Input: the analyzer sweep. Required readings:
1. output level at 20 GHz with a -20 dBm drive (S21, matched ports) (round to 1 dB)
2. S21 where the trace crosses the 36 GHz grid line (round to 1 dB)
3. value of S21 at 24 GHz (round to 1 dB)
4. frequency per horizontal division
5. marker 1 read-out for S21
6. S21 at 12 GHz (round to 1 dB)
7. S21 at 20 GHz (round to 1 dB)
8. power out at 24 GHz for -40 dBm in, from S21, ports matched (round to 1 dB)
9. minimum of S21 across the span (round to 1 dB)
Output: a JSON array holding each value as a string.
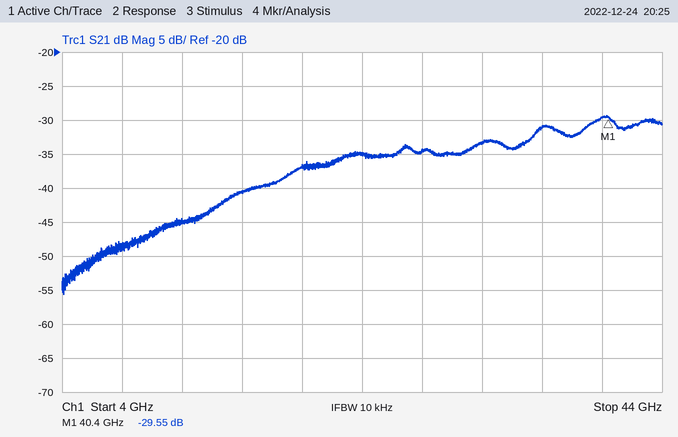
["-57 dBm", "-31 dB", "-35 dB", "4 GHz", "-29.55 dB", "-45 dB", "-37 dB", "-75 dBm", "-56 dB"]
